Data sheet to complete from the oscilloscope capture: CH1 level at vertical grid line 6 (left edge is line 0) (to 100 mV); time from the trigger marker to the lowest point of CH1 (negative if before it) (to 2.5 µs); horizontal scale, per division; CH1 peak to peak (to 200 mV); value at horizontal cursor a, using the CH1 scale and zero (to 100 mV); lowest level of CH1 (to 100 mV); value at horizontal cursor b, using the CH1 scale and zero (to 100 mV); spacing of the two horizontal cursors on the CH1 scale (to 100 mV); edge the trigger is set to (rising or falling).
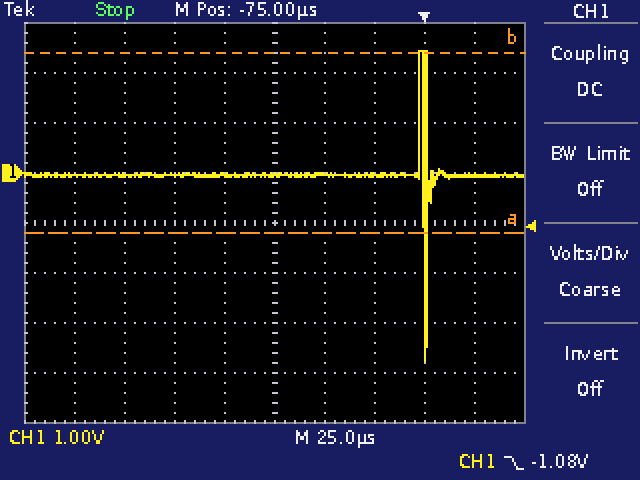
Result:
0.0 V
0.0 µs
25 µs
6.2 V
-1.2 V
-3.8 V
2.4 V
3.6 V
falling
